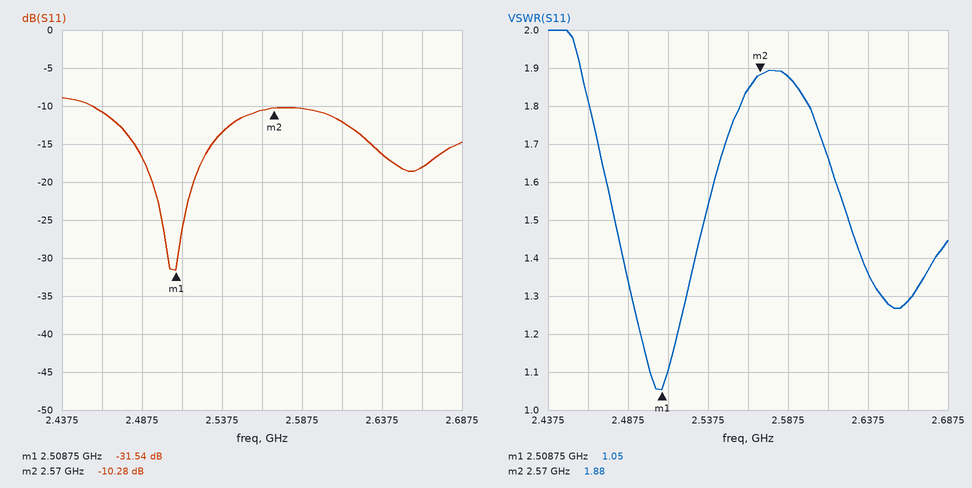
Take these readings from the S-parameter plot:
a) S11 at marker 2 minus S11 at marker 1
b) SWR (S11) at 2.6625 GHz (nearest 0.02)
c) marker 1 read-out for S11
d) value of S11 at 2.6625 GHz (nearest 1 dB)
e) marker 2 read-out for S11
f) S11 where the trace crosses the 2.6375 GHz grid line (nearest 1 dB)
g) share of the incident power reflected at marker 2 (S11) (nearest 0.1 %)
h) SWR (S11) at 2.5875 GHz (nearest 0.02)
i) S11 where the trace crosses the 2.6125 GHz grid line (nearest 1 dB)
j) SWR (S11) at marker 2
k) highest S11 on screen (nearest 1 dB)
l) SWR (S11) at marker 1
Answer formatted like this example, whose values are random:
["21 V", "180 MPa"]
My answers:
["21.26 dB", "1.28", "-31.54 dB", "-18 dB", "-10.28 dB", "-16 dB", "9.4 %", "1.88", "-12 dB", "1.88", "-9 dB", "1.05"]
